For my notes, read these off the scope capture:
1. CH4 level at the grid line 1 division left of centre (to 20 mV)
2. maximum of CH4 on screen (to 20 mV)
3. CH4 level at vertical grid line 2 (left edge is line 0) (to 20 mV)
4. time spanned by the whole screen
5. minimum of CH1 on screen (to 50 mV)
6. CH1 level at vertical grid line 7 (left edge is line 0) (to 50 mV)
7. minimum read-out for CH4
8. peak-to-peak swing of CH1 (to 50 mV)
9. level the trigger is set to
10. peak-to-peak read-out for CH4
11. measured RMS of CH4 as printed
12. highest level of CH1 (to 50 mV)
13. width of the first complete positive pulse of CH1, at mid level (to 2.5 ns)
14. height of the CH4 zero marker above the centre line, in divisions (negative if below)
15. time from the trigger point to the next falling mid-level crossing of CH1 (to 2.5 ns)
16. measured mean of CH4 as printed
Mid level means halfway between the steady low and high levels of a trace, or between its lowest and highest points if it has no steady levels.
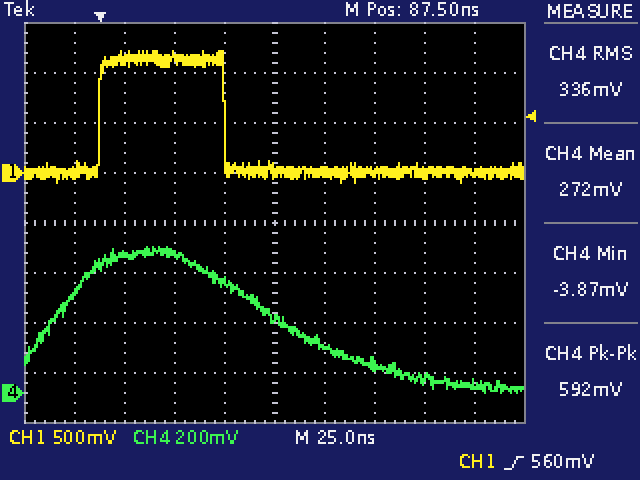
440 mV
580 mV
560 mV
250 ns
-100 mV
0 mV
-3.87 mV
1.30 V
560 mV
592 mV
336 mV
1.20 V
62.5 ns
-3.4 div
62.5 ns
272 mV
